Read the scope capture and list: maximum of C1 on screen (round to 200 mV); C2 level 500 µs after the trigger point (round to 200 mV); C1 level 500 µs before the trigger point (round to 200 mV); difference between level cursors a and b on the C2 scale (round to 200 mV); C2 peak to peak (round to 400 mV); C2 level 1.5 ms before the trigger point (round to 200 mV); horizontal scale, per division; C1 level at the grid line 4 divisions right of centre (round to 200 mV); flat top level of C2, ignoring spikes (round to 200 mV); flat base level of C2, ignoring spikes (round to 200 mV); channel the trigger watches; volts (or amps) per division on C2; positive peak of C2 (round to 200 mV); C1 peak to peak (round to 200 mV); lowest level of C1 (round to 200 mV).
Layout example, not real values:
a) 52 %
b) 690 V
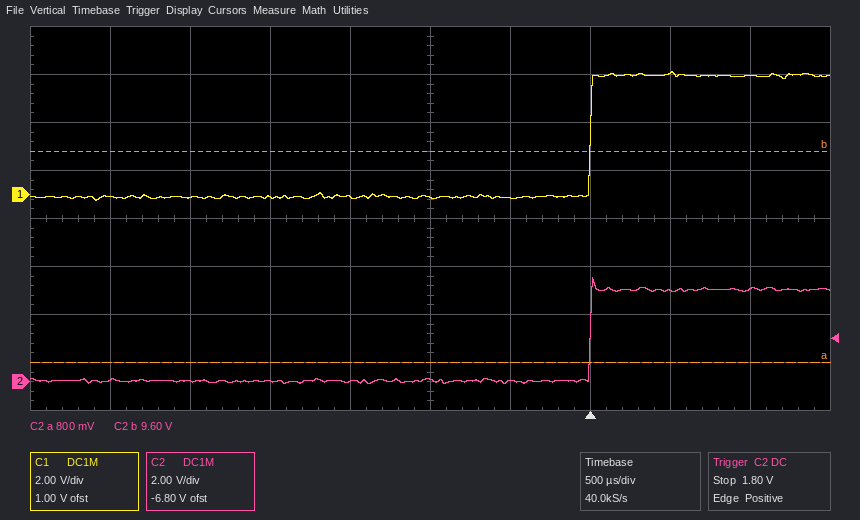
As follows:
a) 5.2 V
b) 3.8 V
c) -200 mV
d) 8.8 V
e) 4.4 V
f) 0.0 V
g) 500 µs
h) 5.0 V
i) 3.8 V
j) 0.0 V
k) C2
l) 2 V
m) 4.4 V
n) 5.4 V
o) -200 mV
